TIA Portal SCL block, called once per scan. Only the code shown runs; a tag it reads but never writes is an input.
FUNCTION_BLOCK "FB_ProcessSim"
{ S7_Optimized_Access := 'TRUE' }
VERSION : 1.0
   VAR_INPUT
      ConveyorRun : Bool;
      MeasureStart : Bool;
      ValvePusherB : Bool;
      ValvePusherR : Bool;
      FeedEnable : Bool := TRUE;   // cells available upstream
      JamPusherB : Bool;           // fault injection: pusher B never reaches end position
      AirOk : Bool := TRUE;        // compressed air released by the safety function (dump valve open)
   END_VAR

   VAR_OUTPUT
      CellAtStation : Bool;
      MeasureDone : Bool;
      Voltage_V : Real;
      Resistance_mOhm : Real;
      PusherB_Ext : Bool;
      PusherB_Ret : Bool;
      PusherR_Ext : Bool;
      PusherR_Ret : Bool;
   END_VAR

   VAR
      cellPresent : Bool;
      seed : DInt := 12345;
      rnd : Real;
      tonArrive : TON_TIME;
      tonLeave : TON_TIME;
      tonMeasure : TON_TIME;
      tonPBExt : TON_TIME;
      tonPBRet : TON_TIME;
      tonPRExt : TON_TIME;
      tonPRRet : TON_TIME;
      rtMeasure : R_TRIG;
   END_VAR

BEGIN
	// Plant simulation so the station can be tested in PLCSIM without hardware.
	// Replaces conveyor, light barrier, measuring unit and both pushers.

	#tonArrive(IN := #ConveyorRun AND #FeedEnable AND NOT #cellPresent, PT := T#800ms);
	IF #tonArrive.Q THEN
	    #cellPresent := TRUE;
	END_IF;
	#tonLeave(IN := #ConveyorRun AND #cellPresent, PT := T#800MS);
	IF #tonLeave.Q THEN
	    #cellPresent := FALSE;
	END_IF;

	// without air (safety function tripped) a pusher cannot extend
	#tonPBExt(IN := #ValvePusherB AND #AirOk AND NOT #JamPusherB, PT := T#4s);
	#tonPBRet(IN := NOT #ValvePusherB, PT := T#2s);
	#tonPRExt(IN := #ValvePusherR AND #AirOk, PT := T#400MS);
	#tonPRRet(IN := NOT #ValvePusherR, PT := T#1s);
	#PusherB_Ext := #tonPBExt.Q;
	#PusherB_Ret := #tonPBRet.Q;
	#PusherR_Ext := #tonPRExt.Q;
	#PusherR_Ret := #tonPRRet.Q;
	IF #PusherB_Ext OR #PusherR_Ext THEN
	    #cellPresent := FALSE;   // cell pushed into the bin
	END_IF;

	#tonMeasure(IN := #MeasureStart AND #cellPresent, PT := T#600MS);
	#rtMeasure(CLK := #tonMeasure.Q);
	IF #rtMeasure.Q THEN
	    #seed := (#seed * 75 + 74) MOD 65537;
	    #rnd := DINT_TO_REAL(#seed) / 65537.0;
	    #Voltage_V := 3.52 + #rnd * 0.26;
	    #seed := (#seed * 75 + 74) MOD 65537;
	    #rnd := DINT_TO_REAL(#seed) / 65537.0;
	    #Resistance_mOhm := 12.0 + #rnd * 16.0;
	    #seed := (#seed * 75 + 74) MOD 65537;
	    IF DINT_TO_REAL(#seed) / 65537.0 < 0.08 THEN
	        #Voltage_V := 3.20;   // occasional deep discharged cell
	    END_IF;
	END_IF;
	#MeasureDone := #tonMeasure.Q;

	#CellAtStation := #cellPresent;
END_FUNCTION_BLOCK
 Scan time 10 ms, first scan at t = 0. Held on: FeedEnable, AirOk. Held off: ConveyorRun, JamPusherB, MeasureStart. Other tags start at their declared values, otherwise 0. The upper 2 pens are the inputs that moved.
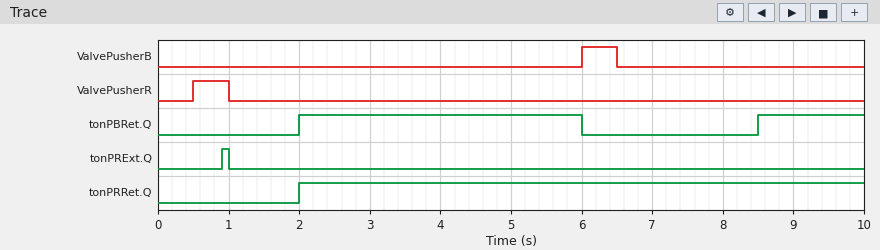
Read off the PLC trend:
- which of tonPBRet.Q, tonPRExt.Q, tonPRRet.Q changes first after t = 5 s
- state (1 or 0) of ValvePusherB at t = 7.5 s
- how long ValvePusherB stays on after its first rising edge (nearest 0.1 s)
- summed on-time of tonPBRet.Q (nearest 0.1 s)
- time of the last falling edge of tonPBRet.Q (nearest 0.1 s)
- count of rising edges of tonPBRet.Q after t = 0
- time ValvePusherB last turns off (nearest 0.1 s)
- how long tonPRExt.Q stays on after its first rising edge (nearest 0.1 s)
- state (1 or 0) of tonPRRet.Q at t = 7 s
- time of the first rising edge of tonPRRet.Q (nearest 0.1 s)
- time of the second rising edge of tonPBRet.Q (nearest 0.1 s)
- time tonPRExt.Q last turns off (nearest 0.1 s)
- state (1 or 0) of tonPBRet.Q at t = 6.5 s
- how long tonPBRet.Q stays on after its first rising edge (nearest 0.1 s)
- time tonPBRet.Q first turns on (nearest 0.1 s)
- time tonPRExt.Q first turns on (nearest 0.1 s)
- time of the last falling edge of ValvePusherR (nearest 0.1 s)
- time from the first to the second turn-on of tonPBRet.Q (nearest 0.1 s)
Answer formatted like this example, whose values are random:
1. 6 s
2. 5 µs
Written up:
1. tonPBRet.Q
2. 0
3. 0.5 s
4. 5.5 s
5. 6.0 s
6. 2
7. 6.5 s
8. 0.1 s
9. 1
10. 2.0 s
11. 8.5 s
12. 1.0 s
13. 0
14. 4.0 s
15. 2.0 s
16. 0.9 s
17. 1.0 s
18. 6.5 s
